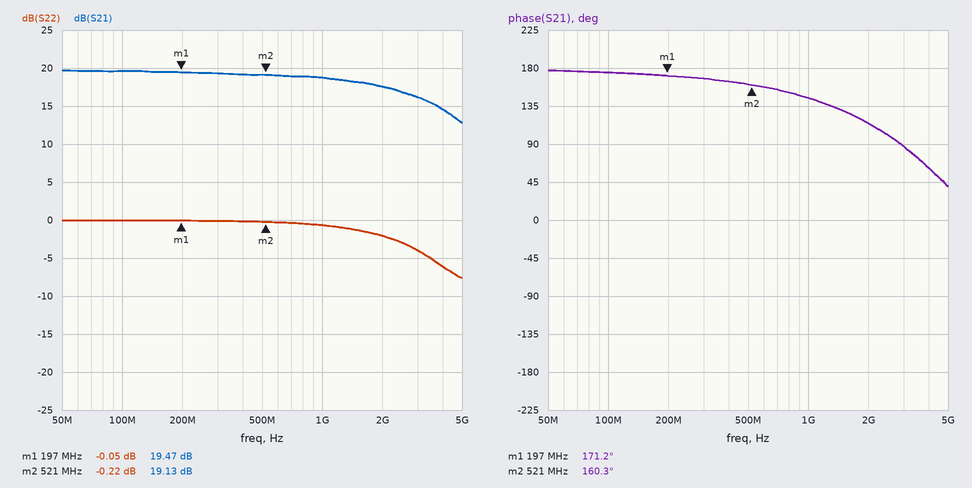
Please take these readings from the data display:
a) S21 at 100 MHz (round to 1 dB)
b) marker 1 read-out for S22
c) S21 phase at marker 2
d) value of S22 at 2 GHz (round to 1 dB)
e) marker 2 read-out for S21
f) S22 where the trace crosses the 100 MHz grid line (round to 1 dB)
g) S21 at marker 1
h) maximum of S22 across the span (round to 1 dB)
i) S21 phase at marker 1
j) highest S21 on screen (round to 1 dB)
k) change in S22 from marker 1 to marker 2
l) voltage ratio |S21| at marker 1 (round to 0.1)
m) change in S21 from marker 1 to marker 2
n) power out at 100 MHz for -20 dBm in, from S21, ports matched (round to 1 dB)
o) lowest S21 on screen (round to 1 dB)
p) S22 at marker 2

20 dB
-0.05 dB
160.3°
-2 dB
19.13 dB
0 dB
19.47 dB
0 dB
171.2°
20 dB
-0.17 dB
9.4
-0.34 dB
0 dBm
13 dB
-0.22 dB
